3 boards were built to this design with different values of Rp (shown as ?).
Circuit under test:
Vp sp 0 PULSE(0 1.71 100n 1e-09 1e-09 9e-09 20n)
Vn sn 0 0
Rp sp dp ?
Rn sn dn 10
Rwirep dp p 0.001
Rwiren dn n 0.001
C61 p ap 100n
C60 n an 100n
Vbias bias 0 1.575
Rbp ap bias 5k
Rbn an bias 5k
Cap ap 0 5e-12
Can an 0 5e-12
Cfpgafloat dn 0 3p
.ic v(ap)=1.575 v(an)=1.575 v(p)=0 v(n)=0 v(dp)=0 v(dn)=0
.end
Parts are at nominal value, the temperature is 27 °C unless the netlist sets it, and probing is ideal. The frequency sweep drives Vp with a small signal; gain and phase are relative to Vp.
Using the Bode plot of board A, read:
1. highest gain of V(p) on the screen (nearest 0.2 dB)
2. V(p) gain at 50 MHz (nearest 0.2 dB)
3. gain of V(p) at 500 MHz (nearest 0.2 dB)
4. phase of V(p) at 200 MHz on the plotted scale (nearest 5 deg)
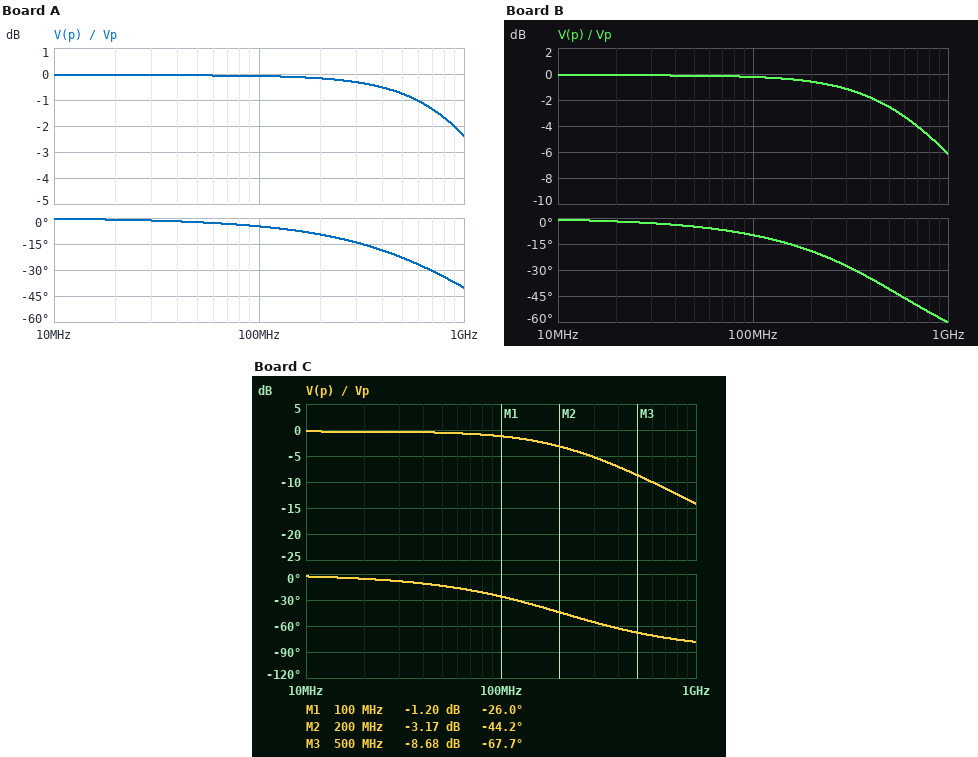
0 dB
0 dB
-0.8 dB
-10 deg
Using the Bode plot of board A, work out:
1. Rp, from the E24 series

27 Ω
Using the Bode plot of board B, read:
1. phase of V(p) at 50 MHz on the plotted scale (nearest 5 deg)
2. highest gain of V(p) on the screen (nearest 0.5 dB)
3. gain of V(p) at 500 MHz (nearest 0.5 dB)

-5 deg
0 dB
-2.5 dB
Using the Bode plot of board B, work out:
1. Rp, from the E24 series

56 Ω
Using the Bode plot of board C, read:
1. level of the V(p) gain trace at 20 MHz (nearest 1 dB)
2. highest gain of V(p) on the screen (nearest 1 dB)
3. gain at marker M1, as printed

0 dB
0 dB
-1.20 dB
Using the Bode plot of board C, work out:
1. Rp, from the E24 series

160 Ω
